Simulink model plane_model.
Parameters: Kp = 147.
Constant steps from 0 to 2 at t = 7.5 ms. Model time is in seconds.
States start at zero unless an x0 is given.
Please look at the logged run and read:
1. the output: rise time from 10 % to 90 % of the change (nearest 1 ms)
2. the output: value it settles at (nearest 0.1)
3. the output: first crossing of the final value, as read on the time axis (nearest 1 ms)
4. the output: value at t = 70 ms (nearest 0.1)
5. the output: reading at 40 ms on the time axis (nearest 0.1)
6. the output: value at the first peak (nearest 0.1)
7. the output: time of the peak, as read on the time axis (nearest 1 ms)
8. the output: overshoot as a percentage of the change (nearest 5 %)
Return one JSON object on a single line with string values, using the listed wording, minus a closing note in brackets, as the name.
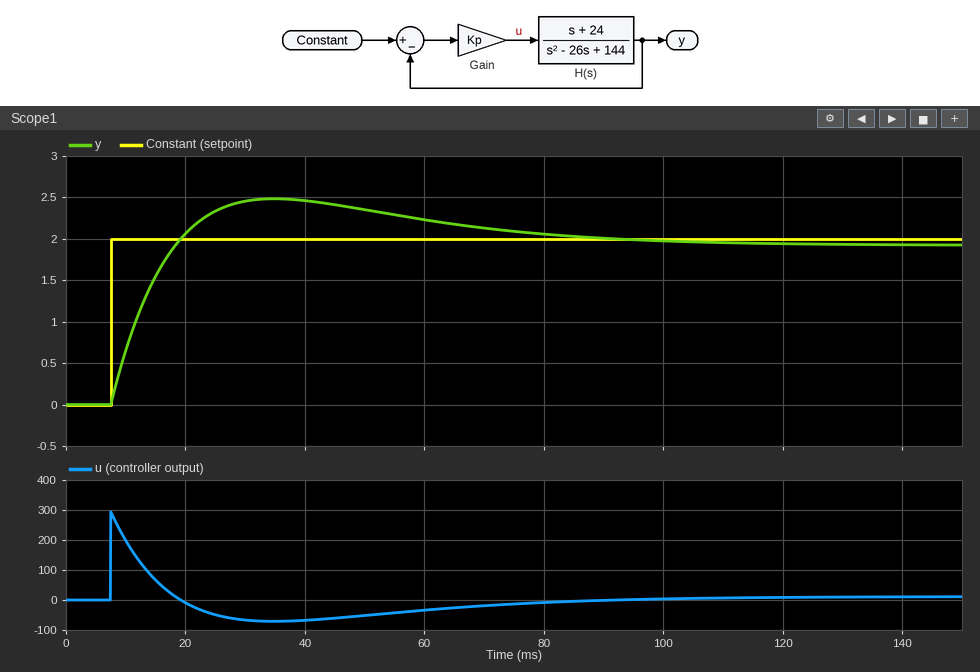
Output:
{"the output: rise time from 10 % to 90 % of the change": "8 ms", "the output: value it settles at": "1.9", "the output: first crossing of the final value, as read on the time axis": "18 ms", "the output: value at t = 70 ms": "2.1", "the output: reading at 40 ms on the time axis": "2.5", "the output: value at the first peak": "2.5", "the output: time of the peak, as read on the time axis": "35 ms", "the output: overshoot as a percentage of the change": "30 %"}
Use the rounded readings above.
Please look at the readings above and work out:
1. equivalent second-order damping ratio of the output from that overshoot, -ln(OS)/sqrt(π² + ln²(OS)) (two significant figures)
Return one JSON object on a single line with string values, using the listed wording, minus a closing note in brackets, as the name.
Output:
{"equivalent second-order damping ratio of the output from that overshoot, -ln(OS)/sqrt(π² + ln²(OS))": "0.36"}
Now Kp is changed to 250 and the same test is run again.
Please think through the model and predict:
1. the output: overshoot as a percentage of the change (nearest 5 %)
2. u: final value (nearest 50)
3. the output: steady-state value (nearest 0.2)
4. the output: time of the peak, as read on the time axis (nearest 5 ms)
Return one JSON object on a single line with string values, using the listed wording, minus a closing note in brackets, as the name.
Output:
{"the output: overshoot as a percentage of the change": "20 %", "u: final value": "0", "the output: steady-state value": "2.0", "the output: time of the peak, as read on the time axis": "25 ms"}
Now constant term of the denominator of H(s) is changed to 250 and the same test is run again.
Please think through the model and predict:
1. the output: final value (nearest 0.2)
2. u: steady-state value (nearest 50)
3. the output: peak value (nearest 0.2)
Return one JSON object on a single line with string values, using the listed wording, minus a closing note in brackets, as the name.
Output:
{"the output: final value": "1.8", "u: steady-state value": "0", "the output: peak value": "2.4"}
